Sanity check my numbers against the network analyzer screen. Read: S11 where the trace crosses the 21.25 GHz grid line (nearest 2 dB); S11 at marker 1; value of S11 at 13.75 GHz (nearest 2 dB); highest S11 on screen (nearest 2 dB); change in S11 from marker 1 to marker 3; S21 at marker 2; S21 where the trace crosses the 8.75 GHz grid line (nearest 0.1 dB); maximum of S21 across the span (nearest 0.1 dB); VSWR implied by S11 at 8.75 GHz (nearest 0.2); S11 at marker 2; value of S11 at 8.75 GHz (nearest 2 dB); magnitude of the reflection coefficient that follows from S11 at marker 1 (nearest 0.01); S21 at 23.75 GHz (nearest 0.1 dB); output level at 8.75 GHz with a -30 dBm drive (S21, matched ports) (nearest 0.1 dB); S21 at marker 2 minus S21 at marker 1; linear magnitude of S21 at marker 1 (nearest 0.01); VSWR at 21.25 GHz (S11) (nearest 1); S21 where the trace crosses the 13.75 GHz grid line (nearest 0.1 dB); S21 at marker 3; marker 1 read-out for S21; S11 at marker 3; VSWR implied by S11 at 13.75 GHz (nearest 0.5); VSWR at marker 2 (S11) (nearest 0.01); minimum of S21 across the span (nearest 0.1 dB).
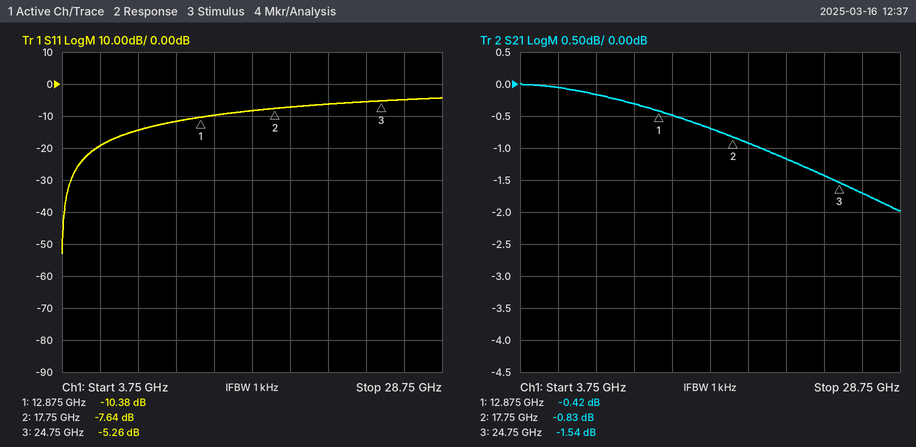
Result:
-6 dB
-10.38 dB
-10 dB
-4 dB
5.12 dB
-0.83 dB
-0.2 dB
0.0 dB
1.4
-7.64 dB
-14 dB
0.30
-1.4 dB
-30.2 dBm
-0.41 dB
0.95
3
-0.5 dB
-1.54 dB
-0.42 dB
-5.26 dB
2.0
2.42
-2.0 dB
